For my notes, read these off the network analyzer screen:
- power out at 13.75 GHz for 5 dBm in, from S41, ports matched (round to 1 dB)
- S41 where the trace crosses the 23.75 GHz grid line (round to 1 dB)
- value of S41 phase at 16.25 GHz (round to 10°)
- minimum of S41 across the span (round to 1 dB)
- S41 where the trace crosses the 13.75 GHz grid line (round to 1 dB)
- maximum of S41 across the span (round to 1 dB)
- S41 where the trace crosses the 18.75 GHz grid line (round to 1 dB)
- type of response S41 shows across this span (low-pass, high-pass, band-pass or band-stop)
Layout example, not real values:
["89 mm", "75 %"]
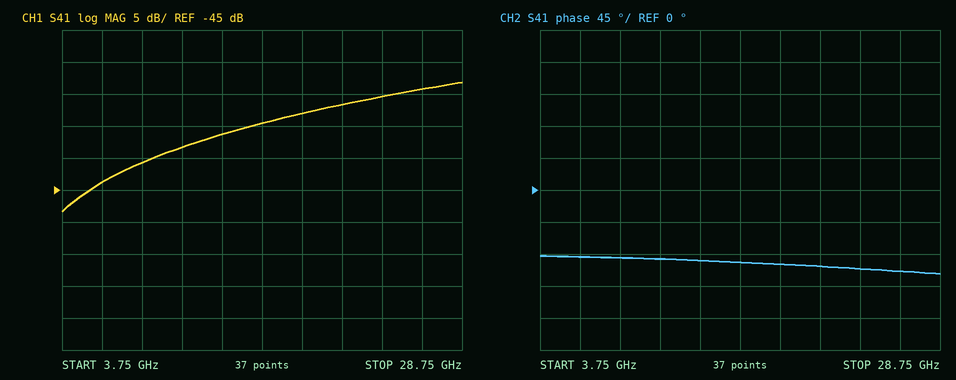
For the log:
["-31 dBm", "-30 dB", "-100°", "-48 dB", "-36 dB", "-28 dB", "-33 dB", "high-pass"]
